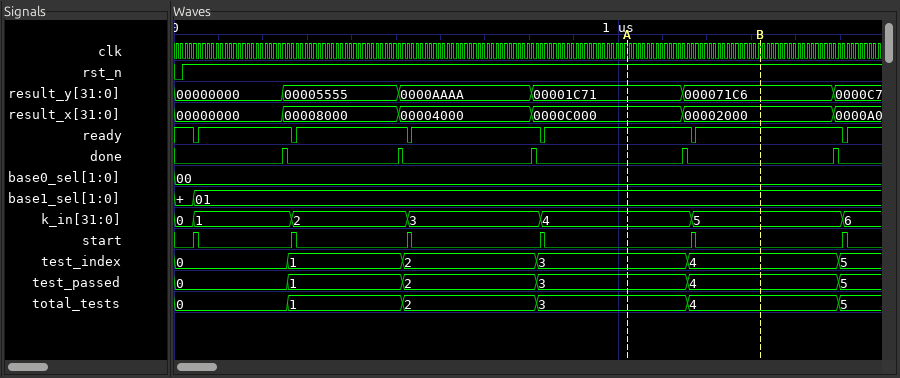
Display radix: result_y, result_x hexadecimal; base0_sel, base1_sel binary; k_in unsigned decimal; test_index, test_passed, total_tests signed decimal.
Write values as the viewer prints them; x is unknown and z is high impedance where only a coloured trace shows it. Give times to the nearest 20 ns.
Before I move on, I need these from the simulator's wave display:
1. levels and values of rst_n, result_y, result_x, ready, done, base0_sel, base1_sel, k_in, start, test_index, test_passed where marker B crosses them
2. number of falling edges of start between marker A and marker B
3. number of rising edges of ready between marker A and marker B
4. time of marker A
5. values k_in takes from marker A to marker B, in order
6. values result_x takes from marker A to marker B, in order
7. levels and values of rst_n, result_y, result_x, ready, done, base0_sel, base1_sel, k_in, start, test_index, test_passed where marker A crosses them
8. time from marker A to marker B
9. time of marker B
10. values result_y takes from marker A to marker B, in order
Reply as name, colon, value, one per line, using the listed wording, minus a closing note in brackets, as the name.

levels and values of rst_n, result_y, result_x, ready, done, base0_sel, base1_sel, k_in, start, test_index, test_passed where marker B crosses them: rst_n=1, result_y=000071C6, result_x=00002000, ready=1, done=0, base0_sel=00, base1_sel=01, k_in=5, start=0, test_index=4, test_passed=4
number of falling edges of start between marker A and marker B: 1
number of rising edges of ready between marker A and marker B: 1
time of marker A: 1020 ns
values k_in takes from marker A to marker B, in order: 4, 5
values result_x takes from marker A to marker B, in order: 0000C000, 00002000
levels and values of rst_n, result_y, result_x, ready, done, base0_sel, base1_sel, k_in, start, test_index, test_passed where marker A crosses them: rst_n=1, result_y=00001C71, result_x=0000C000, ready=1, done=0, base0_sel=00, base1_sel=01, k_in=4, start=0, test_index=3, test_passed=3
time from marker A to marker B: 300 ns
time of marker B: 1320 ns
values result_y takes from marker A to marker B, in order: 00001C71, 000071C6
